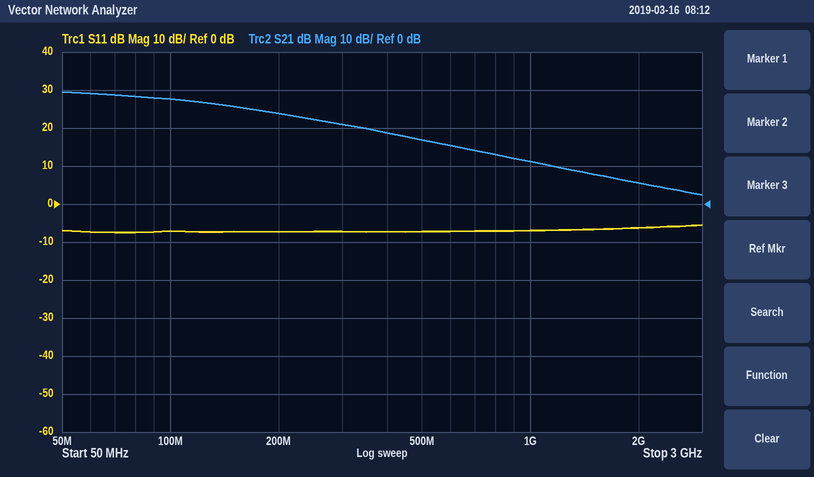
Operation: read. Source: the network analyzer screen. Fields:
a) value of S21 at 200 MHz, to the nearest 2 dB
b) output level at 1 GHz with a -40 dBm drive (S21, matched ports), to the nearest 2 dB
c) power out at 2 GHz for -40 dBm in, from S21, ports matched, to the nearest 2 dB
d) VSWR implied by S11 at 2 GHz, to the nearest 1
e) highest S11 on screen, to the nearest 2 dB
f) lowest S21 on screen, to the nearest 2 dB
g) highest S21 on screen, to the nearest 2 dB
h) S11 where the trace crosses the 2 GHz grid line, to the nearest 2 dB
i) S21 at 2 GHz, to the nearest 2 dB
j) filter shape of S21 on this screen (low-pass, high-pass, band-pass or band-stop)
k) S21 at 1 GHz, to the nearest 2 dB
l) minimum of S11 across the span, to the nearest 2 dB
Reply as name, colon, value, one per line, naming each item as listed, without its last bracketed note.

value of S21 at 200 MHz, to the nearest 2 dB: 24 dB
output level at 1 GHz with a -40 dBm drive (S21, matched ports), to the nearest 2 dB: -28 dBm
power out at 2 GHz for -40 dBm in, from S21, ports matched, to the nearest 2 dB: -34 dBm
VSWR implied by S11 at 2 GHz, to the nearest 1: 3
highest S11 on screen, to the nearest 2 dB: -6 dB
lowest S21 on screen, to the nearest 2 dB: 2 dB
highest S21 on screen, to the nearest 2 dB: 30 dB
S11 where the trace crosses the 2 GHz grid line, to the nearest 2 dB: -6 dB
S21 at 2 GHz, to the nearest 2 dB: 6 dB
filter shape of S21 on this screen: low-pass
S21 at 1 GHz, to the nearest 2 dB: 12 dB
minimum of S11 across the span, to the nearest 2 dB: -8 dB
